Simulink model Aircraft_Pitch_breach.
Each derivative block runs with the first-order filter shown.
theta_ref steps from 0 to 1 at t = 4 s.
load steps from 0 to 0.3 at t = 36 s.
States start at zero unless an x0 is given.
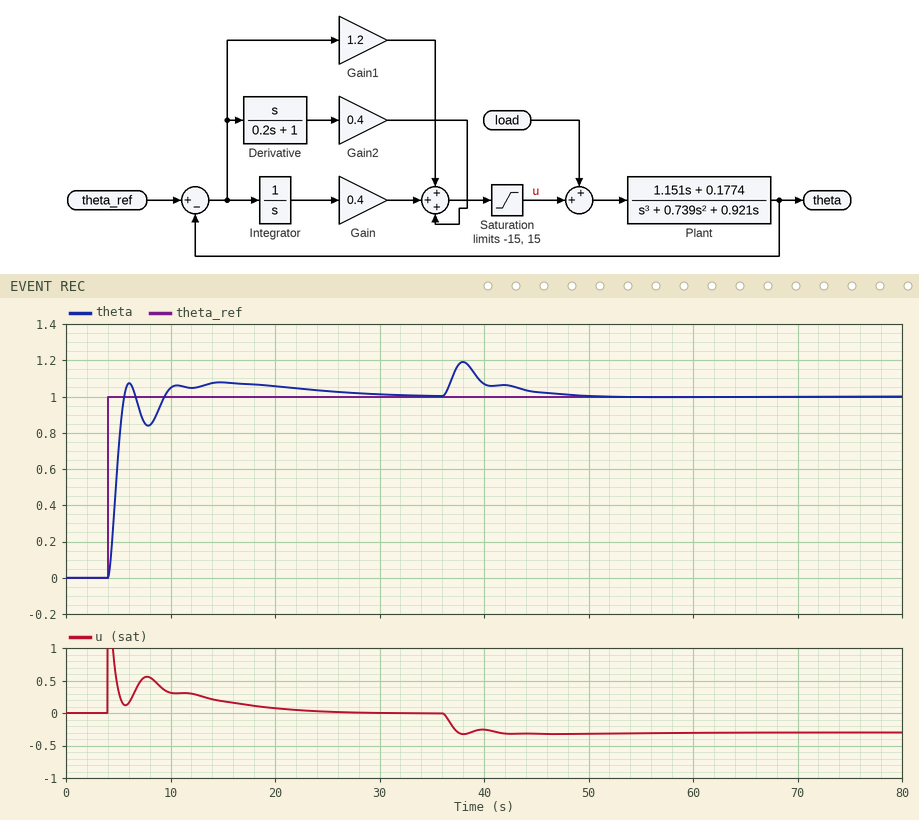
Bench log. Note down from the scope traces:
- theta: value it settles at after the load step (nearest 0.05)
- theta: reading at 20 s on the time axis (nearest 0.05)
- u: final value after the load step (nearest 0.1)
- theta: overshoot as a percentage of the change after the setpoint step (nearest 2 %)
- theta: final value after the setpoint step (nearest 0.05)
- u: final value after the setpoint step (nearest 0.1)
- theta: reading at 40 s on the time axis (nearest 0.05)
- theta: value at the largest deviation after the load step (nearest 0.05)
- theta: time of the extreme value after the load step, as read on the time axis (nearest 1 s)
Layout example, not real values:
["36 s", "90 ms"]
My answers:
["1.00", "1.05", "-0.3", "8 %", "1.00", "0.0", "1.05", "1.20", "38 s"]
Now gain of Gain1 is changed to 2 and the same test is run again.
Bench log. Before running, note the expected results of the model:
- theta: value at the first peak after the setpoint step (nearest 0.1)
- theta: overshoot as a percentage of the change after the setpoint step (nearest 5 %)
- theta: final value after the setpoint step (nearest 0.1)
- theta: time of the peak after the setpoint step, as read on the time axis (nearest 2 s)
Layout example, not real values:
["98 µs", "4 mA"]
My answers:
["1.2", "20 %", "1.0", "6 s"]
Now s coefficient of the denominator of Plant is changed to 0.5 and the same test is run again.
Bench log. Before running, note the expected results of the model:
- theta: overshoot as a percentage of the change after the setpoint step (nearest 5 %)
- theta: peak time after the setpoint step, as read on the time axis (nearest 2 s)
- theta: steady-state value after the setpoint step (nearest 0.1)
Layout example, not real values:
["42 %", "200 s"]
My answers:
["25 %", "6 s", "1.0"]
